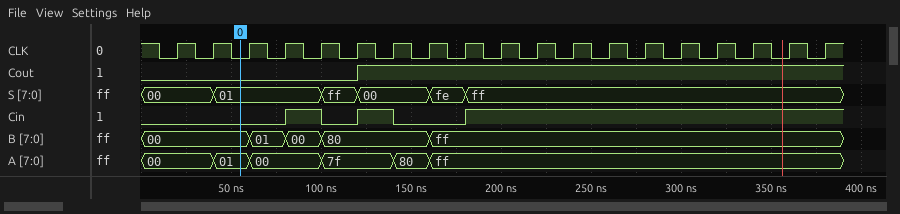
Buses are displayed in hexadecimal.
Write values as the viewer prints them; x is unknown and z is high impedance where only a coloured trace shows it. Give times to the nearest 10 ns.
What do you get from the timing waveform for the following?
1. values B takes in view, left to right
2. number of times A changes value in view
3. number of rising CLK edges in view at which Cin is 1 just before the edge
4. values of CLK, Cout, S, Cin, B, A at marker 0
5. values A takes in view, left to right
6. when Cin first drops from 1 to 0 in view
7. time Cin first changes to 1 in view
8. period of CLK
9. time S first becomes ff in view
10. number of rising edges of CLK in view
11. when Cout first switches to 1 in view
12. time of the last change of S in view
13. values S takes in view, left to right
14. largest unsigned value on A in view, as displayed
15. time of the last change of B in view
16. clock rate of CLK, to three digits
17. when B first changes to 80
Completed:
00, 01, 00, 80, ff
5
12
CLK=0, Cout=0, S=01, Cin=0, B=00, A=01
00, 01, 00, 7f, 80, ff
100 ns
80 ns
20 ns
100 ns
19
120 ns
180 ns
00, 01, ff, 00, fe, ff
ff
160 ns
50.0 MHz
100 ns
